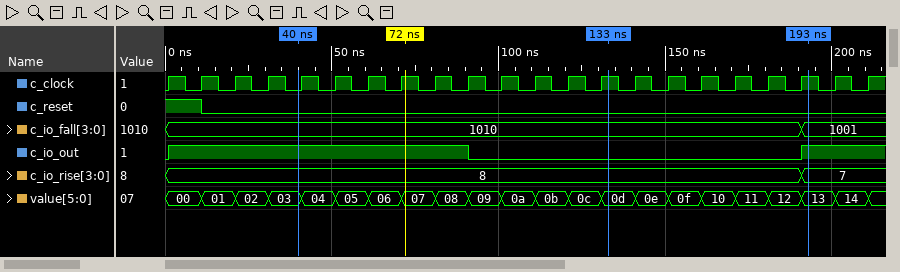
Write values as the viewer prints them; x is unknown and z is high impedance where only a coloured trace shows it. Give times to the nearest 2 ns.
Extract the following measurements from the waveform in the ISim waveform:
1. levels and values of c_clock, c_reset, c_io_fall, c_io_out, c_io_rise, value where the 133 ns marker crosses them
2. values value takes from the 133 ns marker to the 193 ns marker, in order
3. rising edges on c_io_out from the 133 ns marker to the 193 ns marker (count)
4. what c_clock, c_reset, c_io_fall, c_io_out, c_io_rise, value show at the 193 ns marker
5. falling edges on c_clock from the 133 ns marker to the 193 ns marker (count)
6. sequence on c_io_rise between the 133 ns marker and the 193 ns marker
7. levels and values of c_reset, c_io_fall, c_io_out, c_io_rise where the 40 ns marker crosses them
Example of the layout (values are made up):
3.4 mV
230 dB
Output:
c_clock=1, c_reset=0, c_io_fall=1010, c_io_out=0, c_io_rise=8, value=0d
0d, 0e, 0f, 10, 11, 12, 13
1
c_clock=1, c_reset=0, c_io_fall=1001, c_io_out=1, c_io_rise=7, value=13
6
8, 7
c_reset=0, c_io_fall=1010, c_io_out=1, c_io_rise=8
